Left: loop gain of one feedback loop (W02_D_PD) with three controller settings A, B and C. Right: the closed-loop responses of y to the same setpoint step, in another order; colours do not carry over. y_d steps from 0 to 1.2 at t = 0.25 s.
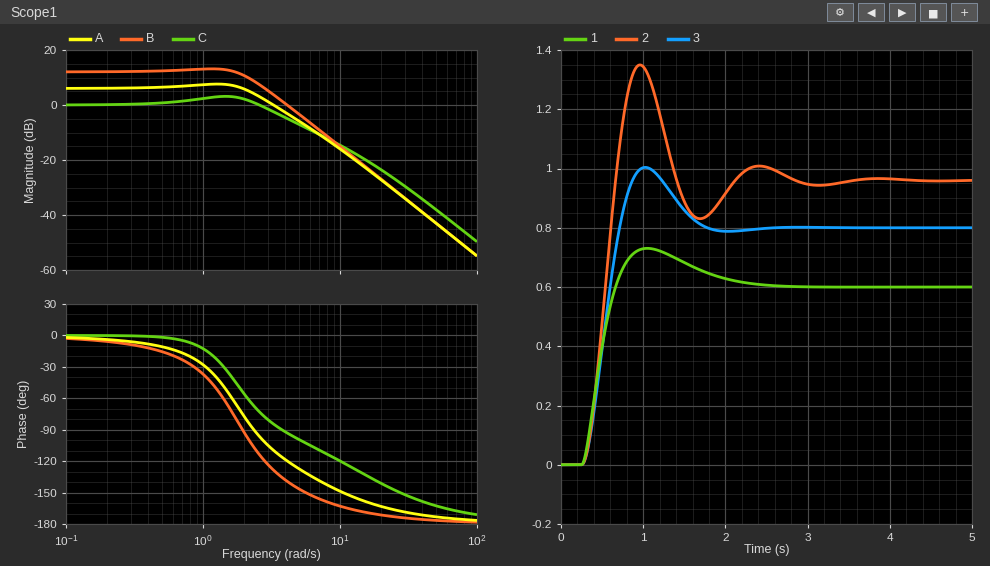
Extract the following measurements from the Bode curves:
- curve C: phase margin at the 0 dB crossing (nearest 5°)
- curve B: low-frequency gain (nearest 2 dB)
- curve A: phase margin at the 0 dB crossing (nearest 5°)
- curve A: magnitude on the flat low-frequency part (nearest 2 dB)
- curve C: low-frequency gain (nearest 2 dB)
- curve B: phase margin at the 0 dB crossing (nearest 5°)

105°
12 dB
70°
6 dB
0 dB
40°
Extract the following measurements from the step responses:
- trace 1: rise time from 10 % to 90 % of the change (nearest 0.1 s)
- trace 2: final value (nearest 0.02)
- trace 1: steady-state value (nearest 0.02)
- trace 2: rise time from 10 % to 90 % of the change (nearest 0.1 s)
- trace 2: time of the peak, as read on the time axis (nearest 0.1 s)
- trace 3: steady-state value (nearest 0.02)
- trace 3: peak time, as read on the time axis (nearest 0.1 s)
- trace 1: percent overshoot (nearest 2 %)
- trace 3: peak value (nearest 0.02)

0.3 s
0.96
0.60
0.3 s
1.0 s
0.80
1.0 s
22 %
1.00
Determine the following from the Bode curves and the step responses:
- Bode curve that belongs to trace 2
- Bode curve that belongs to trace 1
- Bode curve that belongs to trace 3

B
C
A
